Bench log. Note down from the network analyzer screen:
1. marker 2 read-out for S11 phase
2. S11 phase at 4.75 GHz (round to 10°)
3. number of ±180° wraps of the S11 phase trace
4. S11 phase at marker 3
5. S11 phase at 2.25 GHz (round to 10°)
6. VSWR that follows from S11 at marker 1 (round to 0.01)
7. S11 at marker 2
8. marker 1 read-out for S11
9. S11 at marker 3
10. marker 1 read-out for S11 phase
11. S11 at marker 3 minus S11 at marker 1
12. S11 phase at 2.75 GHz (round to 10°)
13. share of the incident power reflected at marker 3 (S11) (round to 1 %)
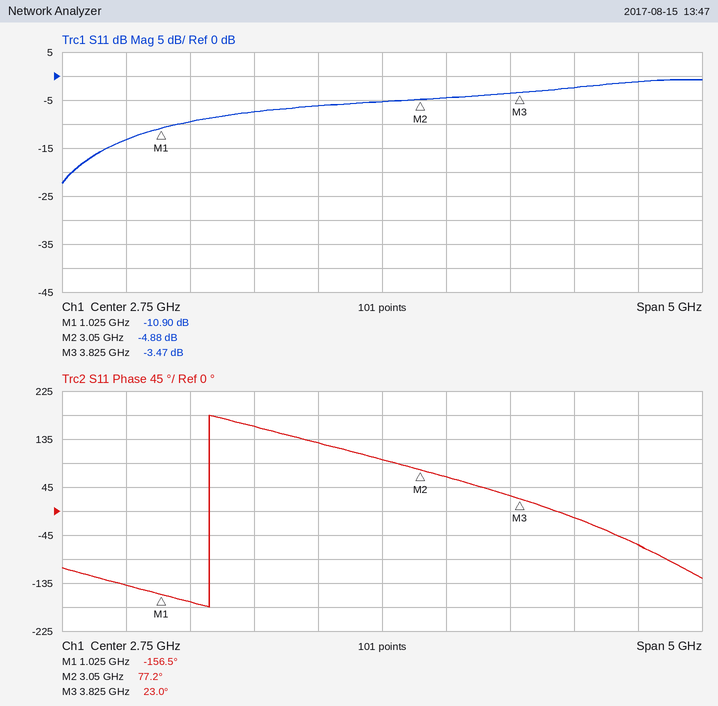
77.2°
-60°
1
23.0°
130°
1.80
-4.88 dB
-10.90 dB
-3.47 dB
-156.5°
7.43 dB
100°
45 %
